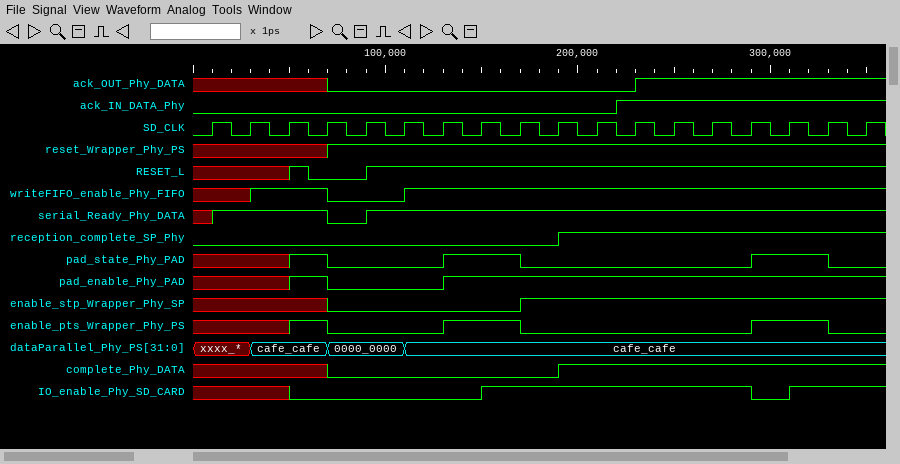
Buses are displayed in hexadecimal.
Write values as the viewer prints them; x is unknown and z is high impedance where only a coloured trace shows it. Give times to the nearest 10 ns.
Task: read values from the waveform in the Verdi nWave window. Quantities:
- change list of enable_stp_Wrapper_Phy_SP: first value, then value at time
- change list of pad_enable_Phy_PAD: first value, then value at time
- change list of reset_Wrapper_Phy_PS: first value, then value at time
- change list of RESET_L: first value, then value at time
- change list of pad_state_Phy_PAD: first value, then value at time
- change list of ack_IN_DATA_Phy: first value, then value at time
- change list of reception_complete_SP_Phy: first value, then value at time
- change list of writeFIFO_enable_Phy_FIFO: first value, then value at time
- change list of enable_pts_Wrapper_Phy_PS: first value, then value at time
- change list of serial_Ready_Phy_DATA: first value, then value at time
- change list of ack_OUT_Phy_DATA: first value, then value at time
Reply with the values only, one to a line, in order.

x, 0 at 70 ns, 1 at 170 ns
x, 1 at 50 ns, 0 at 70 ns, 1 at 130 ns
x, 1 at 70 ns
x, 1 at 50 ns, 0 at 60 ns, 1 at 90 ns
x, 1 at 50 ns, 0 at 70 ns, 1 at 130 ns, 0 at 170 ns, 1 at 290 ns, 0 at 330 ns
0, 1 at 220 ns
0, 1 at 190 ns
x, 1 at 30 ns, 0 at 70 ns, 1 at 110 ns
x, 1 at 50 ns, 0 at 70 ns, 1 at 130 ns, 0 at 170 ns, 1 at 290 ns, 0 at 330 ns
x, 1 at 10 ns, 0 at 70 ns, 1 at 90 ns
x, 0 at 70 ns, 1 at 230 ns
